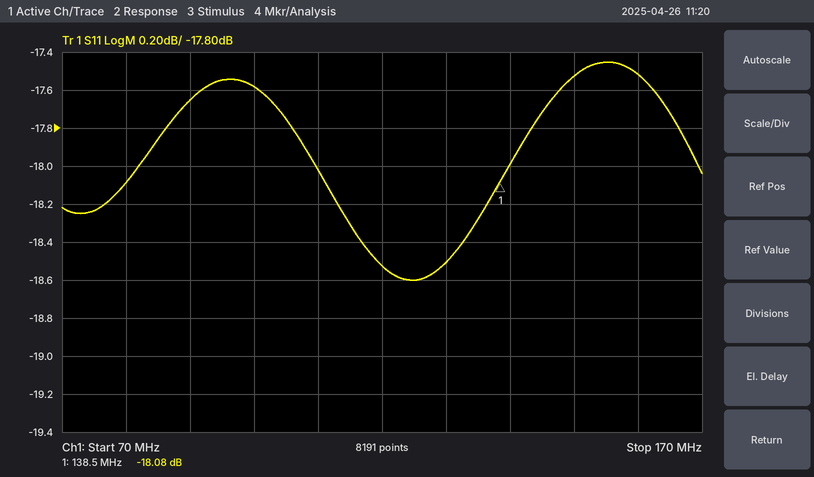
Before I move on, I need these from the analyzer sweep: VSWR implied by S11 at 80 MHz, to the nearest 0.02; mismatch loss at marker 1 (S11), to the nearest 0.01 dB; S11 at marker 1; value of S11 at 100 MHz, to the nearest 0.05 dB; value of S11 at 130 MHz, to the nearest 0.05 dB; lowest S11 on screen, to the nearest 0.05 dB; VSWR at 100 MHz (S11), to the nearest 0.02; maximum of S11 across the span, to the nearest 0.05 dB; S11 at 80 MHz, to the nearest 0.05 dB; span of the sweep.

1.28
0.07 dB
-18.08 dB
-17.60 dB
-18.50 dB
-18.60 dB
1.30
-17.45 dB
-18.10 dB
100 MHz
